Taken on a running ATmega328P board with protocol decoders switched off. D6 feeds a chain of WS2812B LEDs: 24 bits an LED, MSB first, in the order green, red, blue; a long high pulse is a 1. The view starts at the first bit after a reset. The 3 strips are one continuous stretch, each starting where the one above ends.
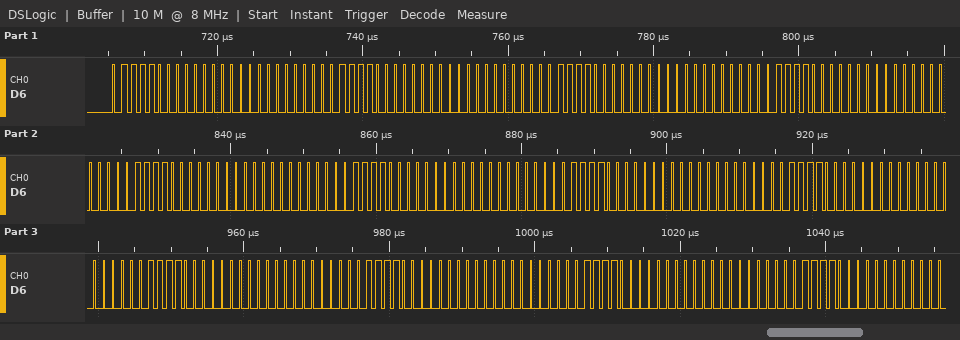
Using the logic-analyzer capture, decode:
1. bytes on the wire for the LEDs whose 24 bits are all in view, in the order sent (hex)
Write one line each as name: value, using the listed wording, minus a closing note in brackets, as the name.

bytes on the wire for the LEDs whose 24 bits are all in view, in the order sent: 78 00 00 78 00 00 78 00 00 78 00 00 78 00 00 78 00 00 78 00 00 78 00 00 78 00 00 78 00 00 78 00 00
